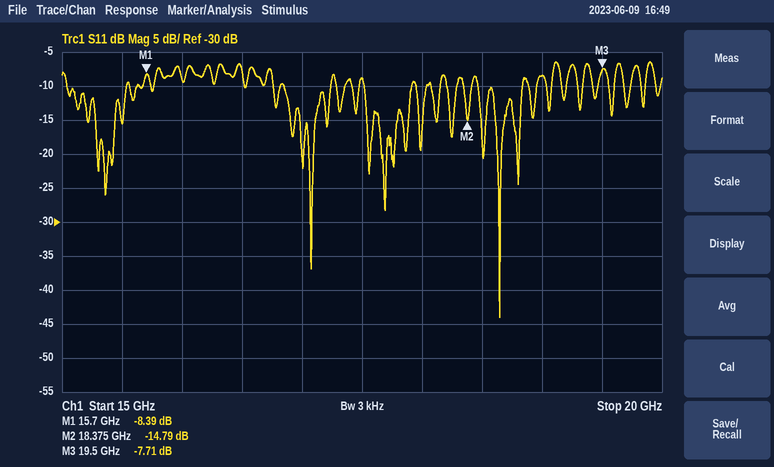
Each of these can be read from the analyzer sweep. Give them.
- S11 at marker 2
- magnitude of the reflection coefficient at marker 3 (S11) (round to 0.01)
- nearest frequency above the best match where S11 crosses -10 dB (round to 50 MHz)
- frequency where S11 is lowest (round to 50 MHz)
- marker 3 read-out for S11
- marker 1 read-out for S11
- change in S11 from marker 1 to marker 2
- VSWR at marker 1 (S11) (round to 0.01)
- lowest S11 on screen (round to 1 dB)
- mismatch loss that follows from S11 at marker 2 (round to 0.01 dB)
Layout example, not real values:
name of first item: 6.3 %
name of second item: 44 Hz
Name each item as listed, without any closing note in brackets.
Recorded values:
S11 at marker 2: -14.79 dB
magnitude of the reflection coefficient at marker 3 (S11): 0.41
nearest frequency above the best match where S11 crosses -10 dB: 18.85 GHz
frequency where S11 is lowest: 18.65 GHz
marker 3 read-out for S11: -7.71 dB
marker 1 read-out for S11: -8.39 dB
change in S11 from marker 1 to marker 2: -6.40 dB
VSWR at marker 1 (S11): 2.23
lowest S11 on screen: -44 dB
mismatch loss that follows from S11 at marker 2: 0.15 dB
